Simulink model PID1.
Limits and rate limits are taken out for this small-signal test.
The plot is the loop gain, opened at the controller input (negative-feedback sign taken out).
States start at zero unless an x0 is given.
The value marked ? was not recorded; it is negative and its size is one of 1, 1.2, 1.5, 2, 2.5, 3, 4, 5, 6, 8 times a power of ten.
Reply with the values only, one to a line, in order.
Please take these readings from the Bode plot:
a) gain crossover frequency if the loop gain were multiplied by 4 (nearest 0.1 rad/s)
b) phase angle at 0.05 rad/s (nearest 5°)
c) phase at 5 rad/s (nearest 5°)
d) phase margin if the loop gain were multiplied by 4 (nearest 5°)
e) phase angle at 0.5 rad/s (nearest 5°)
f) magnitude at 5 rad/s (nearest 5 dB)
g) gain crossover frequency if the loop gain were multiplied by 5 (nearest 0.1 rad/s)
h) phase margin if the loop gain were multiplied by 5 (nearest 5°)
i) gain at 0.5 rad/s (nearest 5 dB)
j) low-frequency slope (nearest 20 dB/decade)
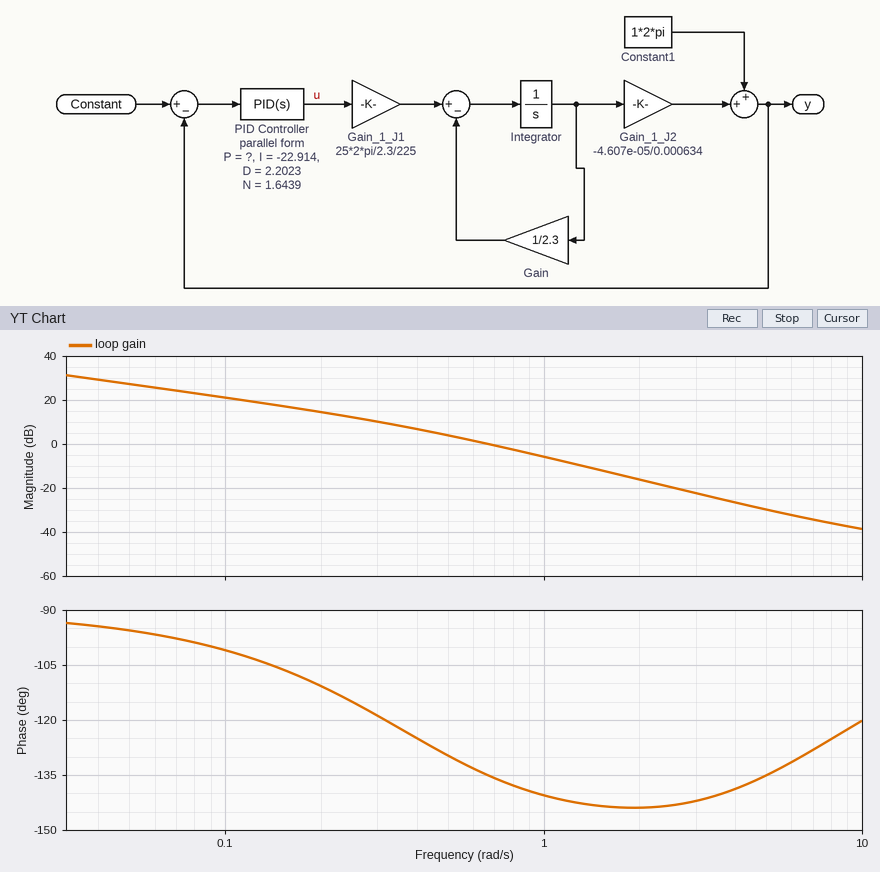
1.5 rad/s
-95°
-135°
35°
-130°
-30 dB
1.7 rad/s
35°
5 dB
-20 dB/decade
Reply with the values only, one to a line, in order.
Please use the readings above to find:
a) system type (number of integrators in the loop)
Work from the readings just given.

1
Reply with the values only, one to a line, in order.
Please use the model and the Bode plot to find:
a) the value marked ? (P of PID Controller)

-8
